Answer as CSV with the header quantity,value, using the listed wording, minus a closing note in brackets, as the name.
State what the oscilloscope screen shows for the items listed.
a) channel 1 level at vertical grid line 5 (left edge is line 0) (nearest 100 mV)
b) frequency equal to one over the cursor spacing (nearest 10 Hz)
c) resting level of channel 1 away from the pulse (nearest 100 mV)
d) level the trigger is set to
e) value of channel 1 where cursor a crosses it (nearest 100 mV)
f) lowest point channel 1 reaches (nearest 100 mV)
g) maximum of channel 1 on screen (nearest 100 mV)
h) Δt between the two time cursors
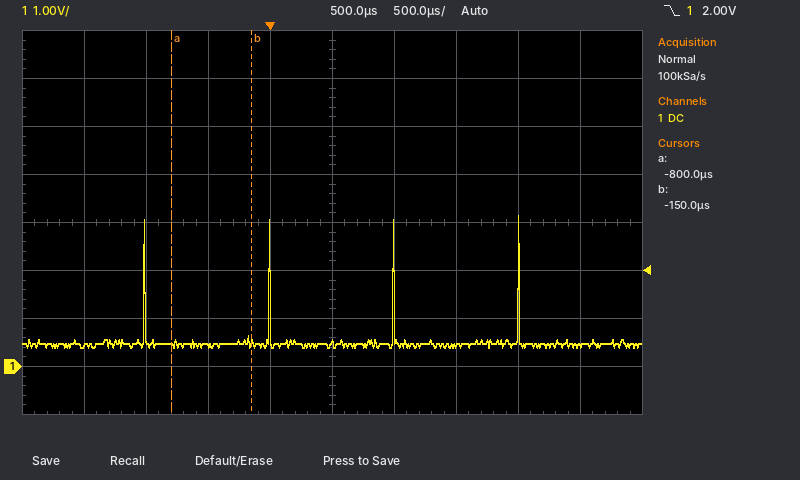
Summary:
quantity,value
channel 1 level at vertical grid line 5 (left edge is line 0),500 mV
frequency equal to one over the cursor spacing,1.54 kHz
resting level of channel 1 away from the pulse,500 mV
level the trigger is set to,2.00 V
value of channel 1 where cursor a crosses it,500 mV
lowest point channel 1 reaches,400 mV
maximum of channel 1 on screen,3.1 V
Δt between the two time cursors,650 µs
